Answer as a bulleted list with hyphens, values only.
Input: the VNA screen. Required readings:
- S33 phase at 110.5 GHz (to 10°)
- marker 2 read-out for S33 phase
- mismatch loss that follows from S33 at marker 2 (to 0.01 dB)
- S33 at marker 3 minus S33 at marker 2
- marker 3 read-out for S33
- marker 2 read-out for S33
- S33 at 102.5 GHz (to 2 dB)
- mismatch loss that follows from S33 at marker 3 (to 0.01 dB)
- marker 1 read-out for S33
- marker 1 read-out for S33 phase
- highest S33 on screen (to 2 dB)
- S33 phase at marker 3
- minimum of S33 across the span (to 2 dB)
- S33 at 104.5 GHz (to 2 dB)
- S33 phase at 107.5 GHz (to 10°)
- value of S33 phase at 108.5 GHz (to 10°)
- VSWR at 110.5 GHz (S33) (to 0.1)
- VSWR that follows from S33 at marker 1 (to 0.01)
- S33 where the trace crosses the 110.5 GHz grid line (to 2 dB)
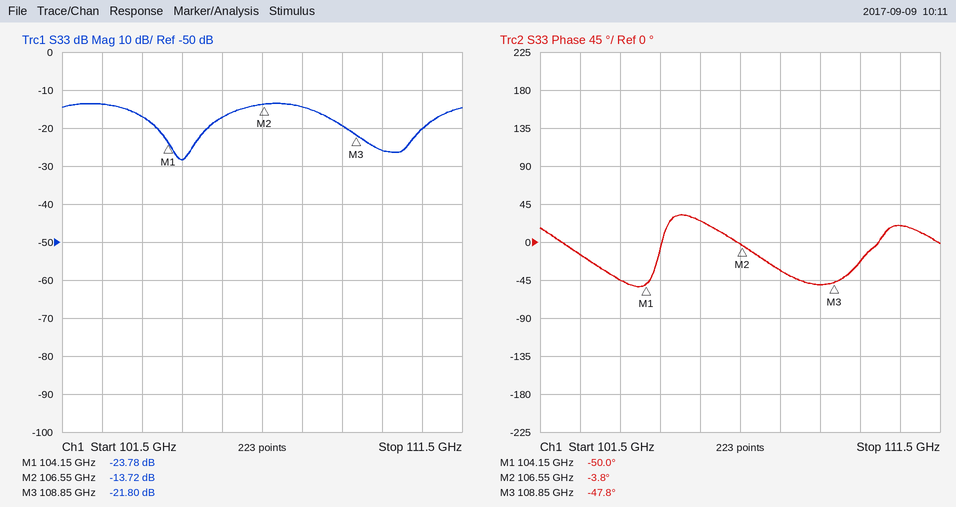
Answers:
- 20°
- -3.8°
- 0.19 dB
- -8.08 dB
- -21.80 dB
- -13.72 dB
- -14 dB
- 0.03 dB
- -23.78 dB
- -50.0°
- -14 dB
- -47.8°
- -28 dB
- -28 dB
- -30°
- -50°
- 1.2
- 1.14
- -20 dB
